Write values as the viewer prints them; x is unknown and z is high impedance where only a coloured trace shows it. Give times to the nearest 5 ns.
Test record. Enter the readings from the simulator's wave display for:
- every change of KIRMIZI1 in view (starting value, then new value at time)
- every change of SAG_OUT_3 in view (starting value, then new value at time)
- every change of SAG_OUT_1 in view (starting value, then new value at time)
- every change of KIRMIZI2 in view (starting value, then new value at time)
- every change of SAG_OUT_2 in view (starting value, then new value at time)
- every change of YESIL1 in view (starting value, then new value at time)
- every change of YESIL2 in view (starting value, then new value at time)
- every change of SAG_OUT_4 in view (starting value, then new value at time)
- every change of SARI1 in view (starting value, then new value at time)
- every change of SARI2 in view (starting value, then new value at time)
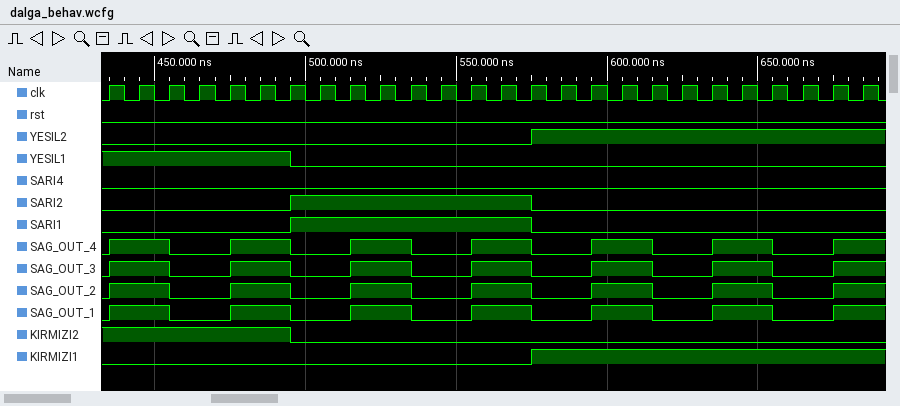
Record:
0, 1 at 575 ns
0, 1 at 435 ns, 0 at 455 ns, 1 at 475 ns, 0 at 495 ns, 1 at 515 ns, 0 at 535 ns, 1 at 555 ns, 0 at 575 ns, 1 at 595 ns, 0 at 615 ns, 1 at 635 ns, 0 at 655 ns, 1 at 675 ns
0, 1 at 435 ns, 0 at 455 ns, 1 at 475 ns, 0 at 495 ns, 1 at 515 ns, 0 at 535 ns, 1 at 555 ns, 0 at 575 ns, 1 at 595 ns, 0 at 615 ns, 1 at 635 ns, 0 at 655 ns, 1 at 675 ns
1, 0 at 495 ns
0, 1 at 435 ns, 0 at 455 ns, 1 at 475 ns, 0 at 495 ns, 1 at 515 ns, 0 at 535 ns, 1 at 555 ns, 0 at 575 ns, 1 at 595 ns, 0 at 615 ns, 1 at 635 ns, 0 at 655 ns, 1 at 675 ns
1, 0 at 495 ns
0, 1 at 575 ns
0, 1 at 435 ns, 0 at 455 ns, 1 at 475 ns, 0 at 495 ns, 1 at 515 ns, 0 at 535 ns, 1 at 555 ns, 0 at 575 ns, 1 at 595 ns, 0 at 615 ns, 1 at 635 ns, 0 at 655 ns, 1 at 675 ns
0, 1 at 495 ns, 0 at 575 ns
0, 1 at 495 ns, 0 at 575 ns
